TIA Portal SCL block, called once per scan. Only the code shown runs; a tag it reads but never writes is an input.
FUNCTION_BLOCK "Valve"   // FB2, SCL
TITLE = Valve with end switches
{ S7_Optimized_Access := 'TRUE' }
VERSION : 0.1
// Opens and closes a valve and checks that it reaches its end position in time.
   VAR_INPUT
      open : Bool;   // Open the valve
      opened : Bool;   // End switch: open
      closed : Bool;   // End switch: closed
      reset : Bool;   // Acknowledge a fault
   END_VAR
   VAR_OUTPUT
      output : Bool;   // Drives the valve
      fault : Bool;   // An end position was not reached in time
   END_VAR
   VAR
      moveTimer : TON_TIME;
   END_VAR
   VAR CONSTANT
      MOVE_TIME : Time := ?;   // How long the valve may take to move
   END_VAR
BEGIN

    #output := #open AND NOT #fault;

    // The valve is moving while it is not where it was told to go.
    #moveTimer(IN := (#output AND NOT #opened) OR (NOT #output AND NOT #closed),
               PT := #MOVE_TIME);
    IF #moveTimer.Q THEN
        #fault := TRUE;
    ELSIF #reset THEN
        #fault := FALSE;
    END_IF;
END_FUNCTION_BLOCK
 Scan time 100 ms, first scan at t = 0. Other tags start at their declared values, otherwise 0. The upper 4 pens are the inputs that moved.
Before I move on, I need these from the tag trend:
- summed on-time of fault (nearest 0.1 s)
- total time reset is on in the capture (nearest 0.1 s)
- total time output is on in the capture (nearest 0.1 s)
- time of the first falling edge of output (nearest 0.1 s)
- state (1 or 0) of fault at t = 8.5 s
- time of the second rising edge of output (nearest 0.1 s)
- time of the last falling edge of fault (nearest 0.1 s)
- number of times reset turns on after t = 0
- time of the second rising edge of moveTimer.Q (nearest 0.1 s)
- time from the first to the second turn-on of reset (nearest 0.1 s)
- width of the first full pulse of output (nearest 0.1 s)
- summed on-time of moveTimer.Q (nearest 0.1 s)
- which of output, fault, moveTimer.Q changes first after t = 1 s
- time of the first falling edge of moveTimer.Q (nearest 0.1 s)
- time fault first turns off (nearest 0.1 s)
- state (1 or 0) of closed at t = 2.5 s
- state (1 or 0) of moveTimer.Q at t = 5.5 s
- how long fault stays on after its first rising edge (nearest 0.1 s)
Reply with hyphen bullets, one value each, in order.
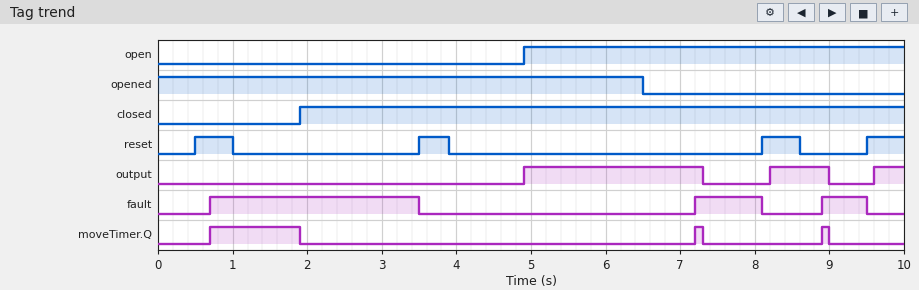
- 4.3 s
- 1.9 s
- 3.6 s
- 7.3 s
- 0
- 8.2 s
- 9.5 s
- 4
- 7.2 s
- 3.0 s
- 2.4 s
- 1.4 s
- moveTimer.Q
- 1.9 s
- 3.5 s
- 1
- 0
- 2.8 s
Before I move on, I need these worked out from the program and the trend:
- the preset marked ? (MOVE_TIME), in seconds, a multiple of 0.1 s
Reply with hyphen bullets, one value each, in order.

- 0.7 s
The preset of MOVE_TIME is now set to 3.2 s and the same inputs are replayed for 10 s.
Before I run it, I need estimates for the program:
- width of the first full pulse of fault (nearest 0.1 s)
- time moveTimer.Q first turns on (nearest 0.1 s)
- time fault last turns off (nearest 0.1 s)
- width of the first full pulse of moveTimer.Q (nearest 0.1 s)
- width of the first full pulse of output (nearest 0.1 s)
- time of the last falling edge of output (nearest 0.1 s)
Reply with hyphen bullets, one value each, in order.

- 0.1 s
- 9.7 s
- 9.8 s
- 0.1 s
- 4.9 s
- 9.8 s
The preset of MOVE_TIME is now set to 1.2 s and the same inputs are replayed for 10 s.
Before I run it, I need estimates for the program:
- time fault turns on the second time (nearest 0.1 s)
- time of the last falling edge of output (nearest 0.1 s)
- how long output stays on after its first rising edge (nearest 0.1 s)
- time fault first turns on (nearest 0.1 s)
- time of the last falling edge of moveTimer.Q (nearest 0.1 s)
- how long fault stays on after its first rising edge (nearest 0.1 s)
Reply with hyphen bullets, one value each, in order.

- 7.7 s
- 9.5 s
- 2.9 s
- 1.2 s
- 9.5 s
- 2.3 s
